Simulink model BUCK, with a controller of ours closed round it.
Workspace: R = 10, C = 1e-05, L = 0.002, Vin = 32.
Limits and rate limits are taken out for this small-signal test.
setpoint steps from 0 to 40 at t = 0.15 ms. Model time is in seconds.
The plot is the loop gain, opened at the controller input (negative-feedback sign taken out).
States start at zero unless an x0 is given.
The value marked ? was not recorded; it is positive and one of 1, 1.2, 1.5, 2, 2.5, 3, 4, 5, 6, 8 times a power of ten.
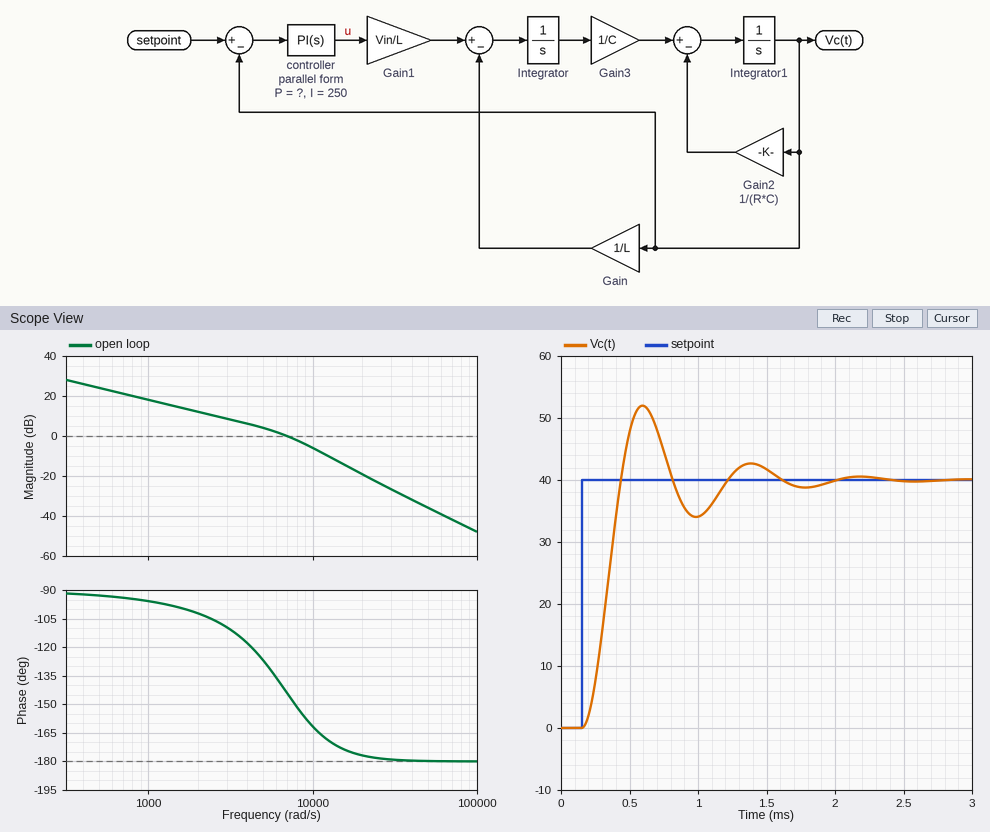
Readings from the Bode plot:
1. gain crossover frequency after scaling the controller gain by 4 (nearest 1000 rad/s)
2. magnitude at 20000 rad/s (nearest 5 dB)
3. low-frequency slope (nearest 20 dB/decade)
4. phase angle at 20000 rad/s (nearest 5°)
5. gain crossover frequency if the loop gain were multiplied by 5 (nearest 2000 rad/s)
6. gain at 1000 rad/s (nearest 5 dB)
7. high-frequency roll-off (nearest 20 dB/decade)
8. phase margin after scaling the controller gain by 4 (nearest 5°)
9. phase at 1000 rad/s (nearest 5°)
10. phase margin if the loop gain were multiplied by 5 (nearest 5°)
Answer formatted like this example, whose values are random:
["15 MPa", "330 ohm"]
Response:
["14000 rad/s", "-20 dB", "-20 dB/decade", "-175°", "16000 rad/s", "20 dB", "-40 dB/decade", "10°", "-95°", "5°"]
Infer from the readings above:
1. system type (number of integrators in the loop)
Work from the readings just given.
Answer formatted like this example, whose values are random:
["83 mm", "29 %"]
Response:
["1"]
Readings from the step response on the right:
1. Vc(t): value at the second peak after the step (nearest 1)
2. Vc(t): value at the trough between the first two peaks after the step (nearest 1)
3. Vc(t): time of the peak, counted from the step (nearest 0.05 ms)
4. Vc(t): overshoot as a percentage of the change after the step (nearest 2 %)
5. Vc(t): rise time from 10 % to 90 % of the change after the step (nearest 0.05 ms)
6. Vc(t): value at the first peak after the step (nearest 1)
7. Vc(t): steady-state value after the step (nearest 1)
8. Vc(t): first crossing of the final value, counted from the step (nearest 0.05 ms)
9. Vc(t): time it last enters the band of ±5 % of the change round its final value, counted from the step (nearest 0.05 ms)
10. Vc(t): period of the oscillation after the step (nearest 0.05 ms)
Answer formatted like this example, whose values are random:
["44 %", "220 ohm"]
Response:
["43", "34", "0.45 ms", "30 %", "0.20 ms", "52", "40", "0.30 ms", "1.35 ms", "0.80 ms"]
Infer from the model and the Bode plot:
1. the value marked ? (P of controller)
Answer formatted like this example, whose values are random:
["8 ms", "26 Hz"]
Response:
["0.025"]
